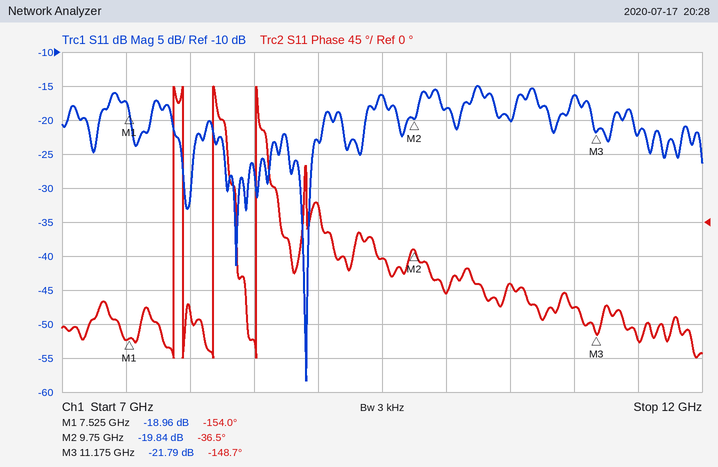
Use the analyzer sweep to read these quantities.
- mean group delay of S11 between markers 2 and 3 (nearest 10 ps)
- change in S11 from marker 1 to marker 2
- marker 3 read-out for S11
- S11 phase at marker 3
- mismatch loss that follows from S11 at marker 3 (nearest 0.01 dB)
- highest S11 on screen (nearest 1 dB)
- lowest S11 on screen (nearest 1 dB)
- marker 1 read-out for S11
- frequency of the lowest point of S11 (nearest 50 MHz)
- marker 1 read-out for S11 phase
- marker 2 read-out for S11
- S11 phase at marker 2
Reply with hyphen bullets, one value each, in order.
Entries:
- 220 ps
- -0.88 dB
- -21.79 dB
- -148.7°
- 0.03 dB
- -15 dB
- -58 dB
- -18.96 dB
- 8.90 GHz
- -154.0°
- -19.84 dB
- -36.5°
